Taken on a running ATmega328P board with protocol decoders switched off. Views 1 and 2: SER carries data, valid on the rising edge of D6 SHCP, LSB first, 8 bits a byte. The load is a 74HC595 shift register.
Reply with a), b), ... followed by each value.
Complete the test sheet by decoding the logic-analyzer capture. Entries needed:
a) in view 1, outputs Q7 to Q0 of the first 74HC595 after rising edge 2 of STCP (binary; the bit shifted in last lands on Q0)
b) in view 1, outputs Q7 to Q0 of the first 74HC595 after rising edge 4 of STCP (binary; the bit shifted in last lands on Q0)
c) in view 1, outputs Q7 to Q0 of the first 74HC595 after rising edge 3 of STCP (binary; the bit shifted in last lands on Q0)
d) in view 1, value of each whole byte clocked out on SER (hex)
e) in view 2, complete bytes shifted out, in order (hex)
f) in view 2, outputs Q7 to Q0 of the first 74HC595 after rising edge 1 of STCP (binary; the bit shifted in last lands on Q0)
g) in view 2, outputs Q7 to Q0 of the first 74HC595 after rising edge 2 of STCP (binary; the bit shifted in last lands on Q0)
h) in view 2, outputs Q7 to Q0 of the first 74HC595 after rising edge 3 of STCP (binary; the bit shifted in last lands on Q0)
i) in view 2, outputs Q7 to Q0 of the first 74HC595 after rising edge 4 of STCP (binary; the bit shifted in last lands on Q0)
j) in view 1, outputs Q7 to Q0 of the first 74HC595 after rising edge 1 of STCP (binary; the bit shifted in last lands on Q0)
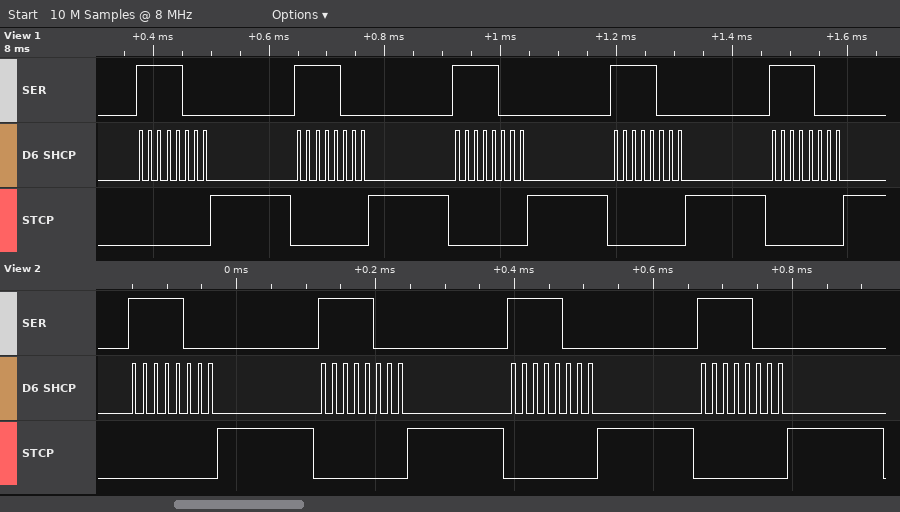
a) 11111000
b) 11111000
c) 11111000
d) 0x1F 0x1F 0x1F 0x1F 0x1F
e) 0x1F 0x1F 0x1F 0x1F
f) 11111000
g) 11111000
h) 11111000
i) 11111000
j) 11111000
